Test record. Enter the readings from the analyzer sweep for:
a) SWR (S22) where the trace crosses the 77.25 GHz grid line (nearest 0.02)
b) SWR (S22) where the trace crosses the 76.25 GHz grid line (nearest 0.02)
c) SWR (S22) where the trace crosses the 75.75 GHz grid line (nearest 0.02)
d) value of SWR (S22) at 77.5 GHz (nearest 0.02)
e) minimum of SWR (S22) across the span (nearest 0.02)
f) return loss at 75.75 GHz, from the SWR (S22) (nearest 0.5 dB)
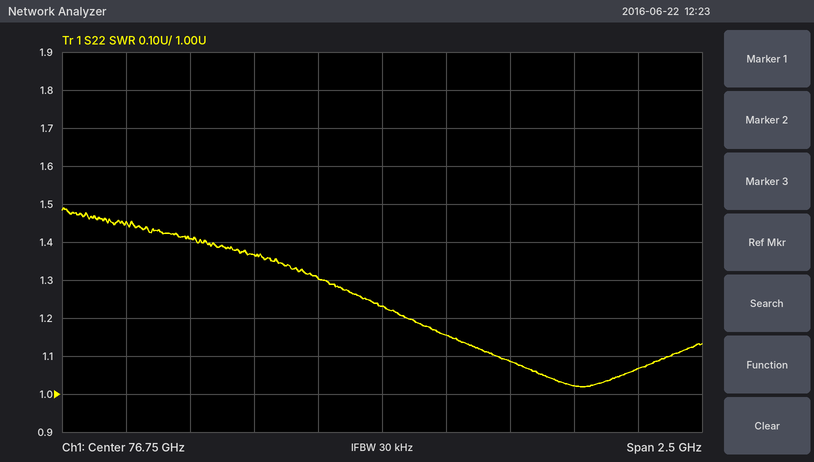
1.08
1.36
1.46
1.02
1.02
14.5 dB
